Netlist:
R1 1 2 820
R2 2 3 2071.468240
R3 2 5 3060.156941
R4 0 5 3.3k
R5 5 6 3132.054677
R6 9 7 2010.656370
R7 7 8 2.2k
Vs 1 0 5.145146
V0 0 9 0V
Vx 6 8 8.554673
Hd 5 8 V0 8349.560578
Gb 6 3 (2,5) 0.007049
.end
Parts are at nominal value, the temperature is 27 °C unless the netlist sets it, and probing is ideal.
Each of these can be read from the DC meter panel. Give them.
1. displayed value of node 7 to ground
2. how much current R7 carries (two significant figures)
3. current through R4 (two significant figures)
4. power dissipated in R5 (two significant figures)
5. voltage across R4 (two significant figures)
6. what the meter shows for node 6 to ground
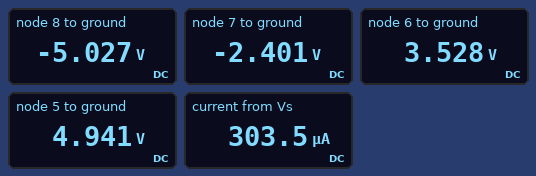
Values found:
-2.401 V
1.2 mA
1.5 mA
640 µW
4.9 V
3.528 V
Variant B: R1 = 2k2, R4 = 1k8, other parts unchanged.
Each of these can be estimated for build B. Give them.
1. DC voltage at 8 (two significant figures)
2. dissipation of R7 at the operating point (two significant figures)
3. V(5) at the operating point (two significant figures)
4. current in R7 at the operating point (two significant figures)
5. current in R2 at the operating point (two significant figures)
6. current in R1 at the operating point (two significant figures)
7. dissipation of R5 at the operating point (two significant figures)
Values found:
-3.2 V
1.3 mW
3.1 V
760 µA
1.0 mA
980 µA
1.6 mW
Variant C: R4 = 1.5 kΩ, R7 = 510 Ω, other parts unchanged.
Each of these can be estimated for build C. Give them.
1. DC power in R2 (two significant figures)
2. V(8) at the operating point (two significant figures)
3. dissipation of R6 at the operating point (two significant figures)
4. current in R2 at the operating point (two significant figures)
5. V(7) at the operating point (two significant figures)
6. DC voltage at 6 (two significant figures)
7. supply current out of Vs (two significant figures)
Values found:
8.3 mW
-1.7 V
880 µW
2.0 mA
-1.3 V
6.9 V
1.9 mA
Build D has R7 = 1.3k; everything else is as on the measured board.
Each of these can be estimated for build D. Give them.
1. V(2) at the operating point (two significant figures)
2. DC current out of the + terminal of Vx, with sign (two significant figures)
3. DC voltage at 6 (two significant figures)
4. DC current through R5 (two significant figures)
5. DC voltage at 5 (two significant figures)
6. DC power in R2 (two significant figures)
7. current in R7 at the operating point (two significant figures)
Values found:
4.7 V
-340 µA
5.4 V
190 µA
4.8 V
580 µW
950 µA
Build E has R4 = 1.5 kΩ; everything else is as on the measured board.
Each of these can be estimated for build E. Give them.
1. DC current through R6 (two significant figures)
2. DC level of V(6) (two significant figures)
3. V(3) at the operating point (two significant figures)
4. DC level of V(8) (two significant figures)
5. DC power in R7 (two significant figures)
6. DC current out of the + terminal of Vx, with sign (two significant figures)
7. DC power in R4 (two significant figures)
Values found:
970 µA
4.5 V
54 mV
-4.1 V
2.1 mW
-1.6 mA
11 mW
